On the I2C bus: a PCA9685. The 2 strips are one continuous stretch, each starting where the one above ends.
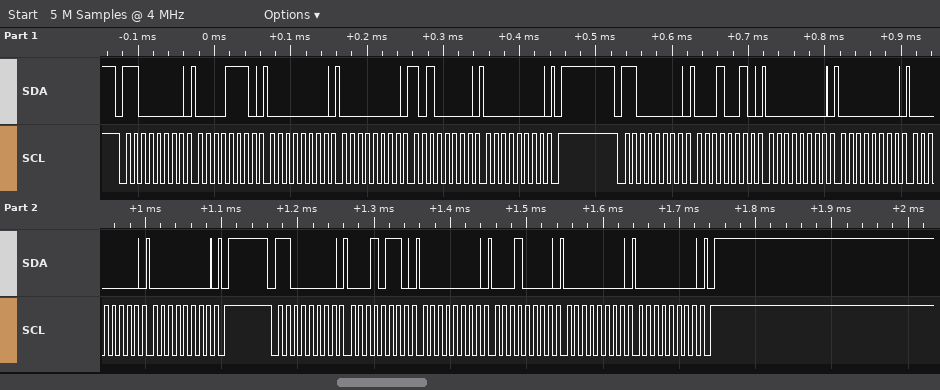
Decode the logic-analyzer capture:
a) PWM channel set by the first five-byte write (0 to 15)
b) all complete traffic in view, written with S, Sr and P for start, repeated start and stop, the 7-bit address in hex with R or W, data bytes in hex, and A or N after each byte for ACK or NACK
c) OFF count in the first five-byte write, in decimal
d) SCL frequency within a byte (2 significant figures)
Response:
2
S 60W A 0E A 00 A 00 A A0 A 00 A P S 60W A 12 A 00 A 00 A 00 A 00 A P S 60W A 16 A 00 A 10 A 00 A 00 A P
160
100 kHz
